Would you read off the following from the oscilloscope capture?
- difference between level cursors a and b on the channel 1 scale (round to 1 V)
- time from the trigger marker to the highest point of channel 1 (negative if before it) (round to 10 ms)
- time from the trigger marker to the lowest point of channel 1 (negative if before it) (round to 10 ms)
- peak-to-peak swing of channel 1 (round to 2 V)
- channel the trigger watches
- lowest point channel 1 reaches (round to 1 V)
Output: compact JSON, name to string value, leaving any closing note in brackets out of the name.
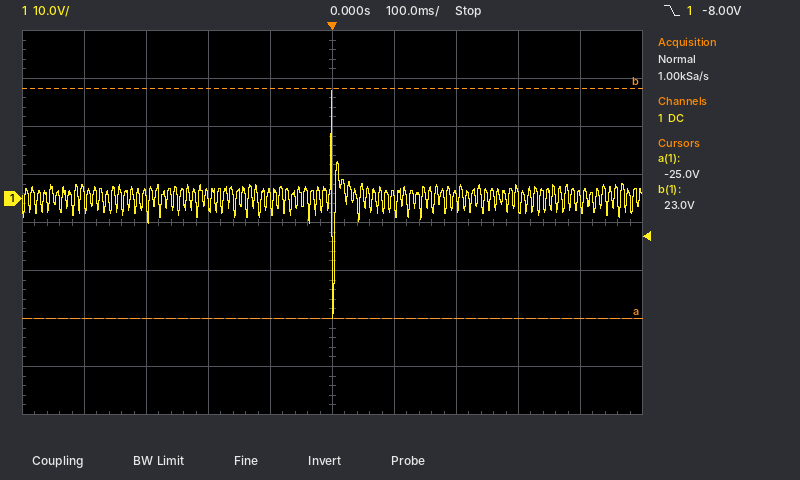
{"difference between level cursors a and b on the channel 1 scale": "48 V", "time from the trigger marker to the highest point of channel 1 (negative if before it)": "0 ms", "time from the trigger marker to the lowest point of channel 1 (negative if before it)": "0 ms", "peak-to-peak swing of channel 1": "48 V", "channel the trigger watches": "channel 1", "lowest point channel 1 reaches": "-25 V"}
